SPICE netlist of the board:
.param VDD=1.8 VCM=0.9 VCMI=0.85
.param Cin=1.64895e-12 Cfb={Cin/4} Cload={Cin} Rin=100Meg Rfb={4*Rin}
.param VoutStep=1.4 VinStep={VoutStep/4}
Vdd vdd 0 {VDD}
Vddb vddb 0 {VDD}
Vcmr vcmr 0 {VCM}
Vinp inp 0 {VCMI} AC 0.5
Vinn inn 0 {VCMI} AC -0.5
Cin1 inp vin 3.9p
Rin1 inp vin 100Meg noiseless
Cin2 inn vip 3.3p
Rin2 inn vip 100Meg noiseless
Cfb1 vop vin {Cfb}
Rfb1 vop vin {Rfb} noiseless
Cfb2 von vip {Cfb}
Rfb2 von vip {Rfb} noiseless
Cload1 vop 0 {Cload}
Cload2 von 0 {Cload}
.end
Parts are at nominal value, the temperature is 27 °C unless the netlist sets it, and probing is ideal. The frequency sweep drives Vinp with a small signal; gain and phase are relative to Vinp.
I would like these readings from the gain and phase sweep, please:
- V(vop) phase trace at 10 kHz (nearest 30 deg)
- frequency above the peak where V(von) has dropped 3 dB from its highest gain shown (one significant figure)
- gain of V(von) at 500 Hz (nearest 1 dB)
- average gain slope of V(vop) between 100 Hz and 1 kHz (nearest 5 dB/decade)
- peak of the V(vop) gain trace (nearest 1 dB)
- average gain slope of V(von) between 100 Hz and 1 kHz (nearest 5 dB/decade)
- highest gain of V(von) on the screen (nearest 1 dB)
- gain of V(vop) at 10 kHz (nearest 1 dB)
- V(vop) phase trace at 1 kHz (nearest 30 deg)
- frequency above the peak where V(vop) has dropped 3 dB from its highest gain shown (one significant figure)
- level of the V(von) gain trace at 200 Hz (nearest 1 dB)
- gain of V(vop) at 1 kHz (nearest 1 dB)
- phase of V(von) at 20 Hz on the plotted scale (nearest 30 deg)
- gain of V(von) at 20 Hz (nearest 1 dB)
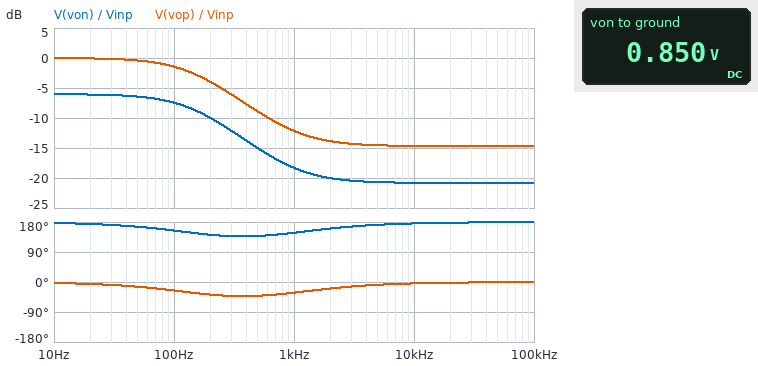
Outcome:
0 deg
200 Hz
-15 dB
-10 dB/decade
0 dB
-10 dB/decade
-6 dB
-15 dB
-30 deg
200 Hz
-10 dB
-12 dB
180 deg
-6 dB
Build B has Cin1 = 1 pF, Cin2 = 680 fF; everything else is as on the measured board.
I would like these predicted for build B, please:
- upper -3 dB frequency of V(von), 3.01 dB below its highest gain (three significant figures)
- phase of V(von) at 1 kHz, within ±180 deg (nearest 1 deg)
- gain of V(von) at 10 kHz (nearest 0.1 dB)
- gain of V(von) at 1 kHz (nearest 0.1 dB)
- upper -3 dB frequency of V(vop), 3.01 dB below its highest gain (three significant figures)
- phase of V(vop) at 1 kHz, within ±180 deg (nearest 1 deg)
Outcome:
168 Hz
140 deg
-23.3 dB
-19.1 dB
167 Hz
-38 deg
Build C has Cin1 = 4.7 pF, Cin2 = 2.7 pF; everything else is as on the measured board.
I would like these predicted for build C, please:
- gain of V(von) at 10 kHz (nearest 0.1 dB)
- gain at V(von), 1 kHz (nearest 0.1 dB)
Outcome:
-21.0 dB
-18.5 dB
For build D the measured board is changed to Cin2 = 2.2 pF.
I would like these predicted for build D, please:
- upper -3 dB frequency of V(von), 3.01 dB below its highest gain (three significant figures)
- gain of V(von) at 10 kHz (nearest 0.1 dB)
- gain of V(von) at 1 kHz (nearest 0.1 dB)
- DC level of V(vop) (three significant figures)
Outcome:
164 Hz
-21.2 dB
-18.6 dB
850 mV
